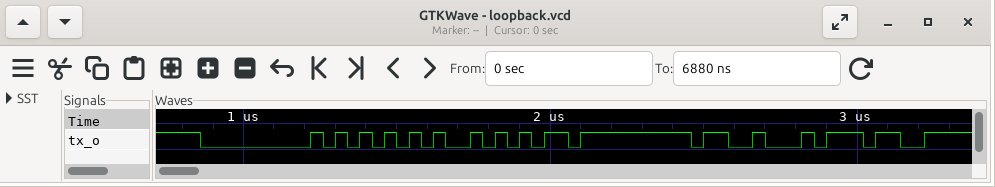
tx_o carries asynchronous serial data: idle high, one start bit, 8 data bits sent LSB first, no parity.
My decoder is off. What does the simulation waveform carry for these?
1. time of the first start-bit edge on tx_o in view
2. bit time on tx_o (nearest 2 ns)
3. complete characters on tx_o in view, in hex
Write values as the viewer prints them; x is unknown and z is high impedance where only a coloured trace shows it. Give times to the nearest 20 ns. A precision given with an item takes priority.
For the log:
860 ns
40 ns
00, 55, AA, FF, 13, 37
